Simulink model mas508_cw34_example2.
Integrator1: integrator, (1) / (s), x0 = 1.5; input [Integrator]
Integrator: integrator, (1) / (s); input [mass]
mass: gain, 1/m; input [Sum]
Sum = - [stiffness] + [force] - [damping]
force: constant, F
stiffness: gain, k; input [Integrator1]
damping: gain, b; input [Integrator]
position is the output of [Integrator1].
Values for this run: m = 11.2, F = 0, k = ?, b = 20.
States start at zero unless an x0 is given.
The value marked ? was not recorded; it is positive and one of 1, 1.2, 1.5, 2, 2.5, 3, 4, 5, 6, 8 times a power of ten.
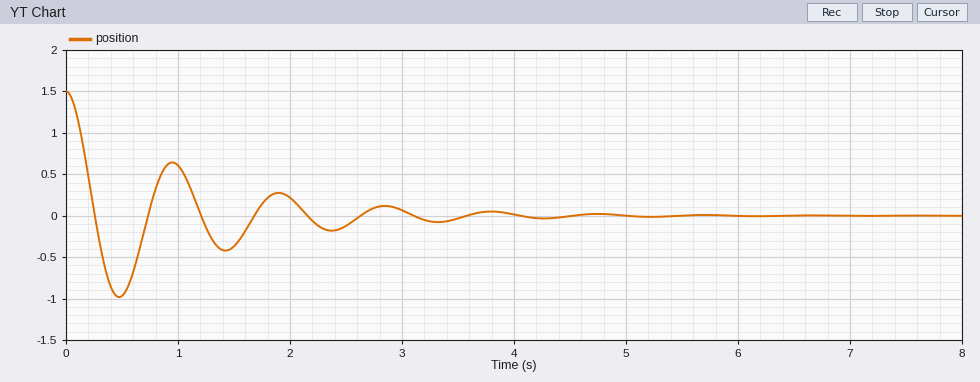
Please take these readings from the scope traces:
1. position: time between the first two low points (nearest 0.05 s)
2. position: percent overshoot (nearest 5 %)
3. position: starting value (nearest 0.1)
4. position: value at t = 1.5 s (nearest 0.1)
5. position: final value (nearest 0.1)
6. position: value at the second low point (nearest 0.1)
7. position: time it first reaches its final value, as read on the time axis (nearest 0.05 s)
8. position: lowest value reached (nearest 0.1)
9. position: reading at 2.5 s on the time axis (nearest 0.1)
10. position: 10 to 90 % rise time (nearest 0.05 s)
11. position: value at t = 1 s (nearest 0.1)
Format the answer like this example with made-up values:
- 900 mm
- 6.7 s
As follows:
- 0.95 s
- 65 %
- 1.5
- -0.4
- 0.0
- -0.4
- 0.25 s
- -1.0
- -0.1
- 0.15 s
- 0.6
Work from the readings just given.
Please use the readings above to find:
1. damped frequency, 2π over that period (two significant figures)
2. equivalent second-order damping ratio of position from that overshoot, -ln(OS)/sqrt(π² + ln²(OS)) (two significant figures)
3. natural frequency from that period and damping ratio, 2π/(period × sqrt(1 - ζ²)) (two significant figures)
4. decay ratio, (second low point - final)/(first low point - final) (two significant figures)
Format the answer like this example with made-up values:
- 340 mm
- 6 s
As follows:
- 6.6 rad/s
- 0.14
- 6.7 rad/s
- 0.40
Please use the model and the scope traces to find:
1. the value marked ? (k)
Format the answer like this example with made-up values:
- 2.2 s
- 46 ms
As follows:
- 500
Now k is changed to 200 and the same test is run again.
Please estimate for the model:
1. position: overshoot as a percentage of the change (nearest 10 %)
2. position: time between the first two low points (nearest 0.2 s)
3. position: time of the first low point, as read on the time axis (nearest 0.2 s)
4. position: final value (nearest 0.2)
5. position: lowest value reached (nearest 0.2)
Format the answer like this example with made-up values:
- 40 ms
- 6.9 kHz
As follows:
- 50 %
- 1.6 s
- 0.8 s
- 0.0
- -0.8
